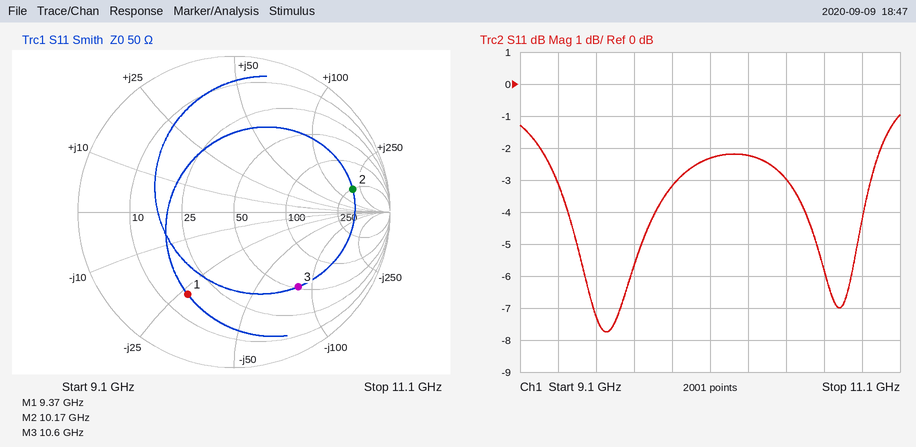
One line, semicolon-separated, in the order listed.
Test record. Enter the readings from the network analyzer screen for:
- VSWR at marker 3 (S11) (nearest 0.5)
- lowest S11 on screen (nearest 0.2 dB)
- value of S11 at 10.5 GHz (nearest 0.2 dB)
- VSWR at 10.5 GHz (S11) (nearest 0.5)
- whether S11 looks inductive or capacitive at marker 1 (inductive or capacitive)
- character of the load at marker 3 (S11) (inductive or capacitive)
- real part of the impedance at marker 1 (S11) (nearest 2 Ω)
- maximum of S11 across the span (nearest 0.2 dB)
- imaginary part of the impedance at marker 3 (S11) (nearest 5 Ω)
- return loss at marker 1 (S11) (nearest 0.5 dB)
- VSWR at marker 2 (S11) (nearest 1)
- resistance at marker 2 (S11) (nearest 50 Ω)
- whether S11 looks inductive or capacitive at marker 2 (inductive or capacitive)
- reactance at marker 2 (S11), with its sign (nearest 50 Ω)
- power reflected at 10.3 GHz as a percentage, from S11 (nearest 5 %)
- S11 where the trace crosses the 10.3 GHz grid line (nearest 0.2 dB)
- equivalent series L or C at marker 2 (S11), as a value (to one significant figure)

4.5; -7.8 dB; -3.0 dB; 6.0; capacitive; capacitive; 16 Ω; -1.0 dB; -85 Ω; 4.5 dB; 8; 250 Ω; inductive; +200 Ω; 60 %; -2.2 dB; 3 nH
